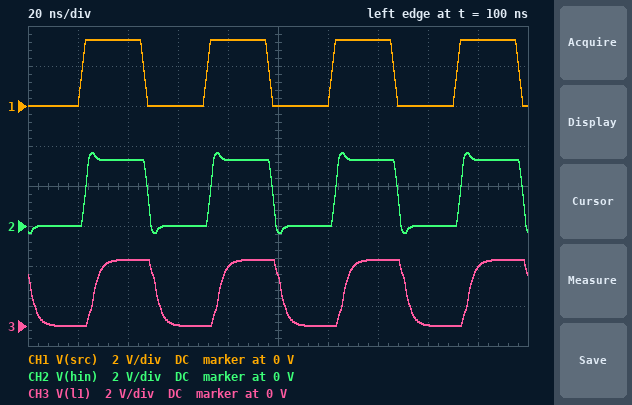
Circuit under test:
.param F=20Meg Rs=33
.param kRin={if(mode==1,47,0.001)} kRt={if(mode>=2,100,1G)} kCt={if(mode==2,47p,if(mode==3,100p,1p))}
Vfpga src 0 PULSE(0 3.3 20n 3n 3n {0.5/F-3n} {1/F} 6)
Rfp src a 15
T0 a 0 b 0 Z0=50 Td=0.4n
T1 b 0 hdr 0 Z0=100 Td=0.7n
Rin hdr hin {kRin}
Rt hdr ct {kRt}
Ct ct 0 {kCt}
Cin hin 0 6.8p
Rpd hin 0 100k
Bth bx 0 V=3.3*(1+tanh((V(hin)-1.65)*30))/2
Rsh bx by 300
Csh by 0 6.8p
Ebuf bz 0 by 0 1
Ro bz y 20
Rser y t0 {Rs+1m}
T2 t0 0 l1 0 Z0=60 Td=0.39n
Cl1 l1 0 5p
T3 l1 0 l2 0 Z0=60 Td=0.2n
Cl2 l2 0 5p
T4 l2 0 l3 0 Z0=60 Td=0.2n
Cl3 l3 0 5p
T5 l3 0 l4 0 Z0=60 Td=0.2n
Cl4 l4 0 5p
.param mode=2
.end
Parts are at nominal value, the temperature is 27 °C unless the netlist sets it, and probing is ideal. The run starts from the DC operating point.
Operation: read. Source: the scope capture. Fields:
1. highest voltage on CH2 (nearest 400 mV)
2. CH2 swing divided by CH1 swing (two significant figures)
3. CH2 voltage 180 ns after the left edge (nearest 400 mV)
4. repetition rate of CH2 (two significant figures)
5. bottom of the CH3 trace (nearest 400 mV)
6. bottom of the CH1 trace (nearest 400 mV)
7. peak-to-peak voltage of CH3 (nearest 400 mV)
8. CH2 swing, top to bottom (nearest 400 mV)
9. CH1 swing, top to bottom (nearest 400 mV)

3.6 V
1.2
3.2 V
20 MHz
0 V
0 V
3.2 V
4.0 V
3.2 V
